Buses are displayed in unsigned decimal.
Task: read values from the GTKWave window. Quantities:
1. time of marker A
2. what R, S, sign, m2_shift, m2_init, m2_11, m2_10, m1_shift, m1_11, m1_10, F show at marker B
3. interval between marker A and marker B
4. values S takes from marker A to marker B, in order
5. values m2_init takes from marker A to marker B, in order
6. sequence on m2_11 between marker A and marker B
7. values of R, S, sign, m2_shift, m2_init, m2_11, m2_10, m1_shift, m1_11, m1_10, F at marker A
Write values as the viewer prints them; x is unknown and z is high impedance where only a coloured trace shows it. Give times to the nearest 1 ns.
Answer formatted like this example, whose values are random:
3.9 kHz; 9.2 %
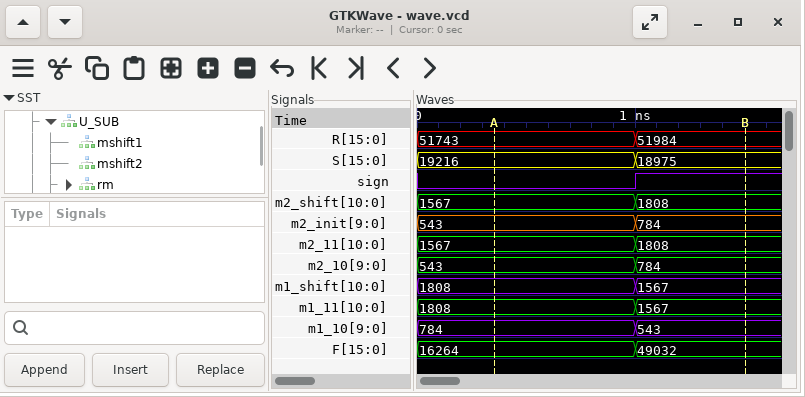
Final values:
0 ns; R=51984, S=18975, sign=1, m2_shift=1808, m2_init=784, m2_11=1808, m2_10=784, m1_shift=1567, m1_11=1567, m1_10=543, F=49032; 1 ns; 19216, 18975; 543, 784; 1567, 1808; R=51743, S=19216, sign=0, m2_shift=1567, m2_init=543, m2_11=1567, m2_10=543, m1_shift=1808, m1_11=1808, m1_10=784, F=16264
